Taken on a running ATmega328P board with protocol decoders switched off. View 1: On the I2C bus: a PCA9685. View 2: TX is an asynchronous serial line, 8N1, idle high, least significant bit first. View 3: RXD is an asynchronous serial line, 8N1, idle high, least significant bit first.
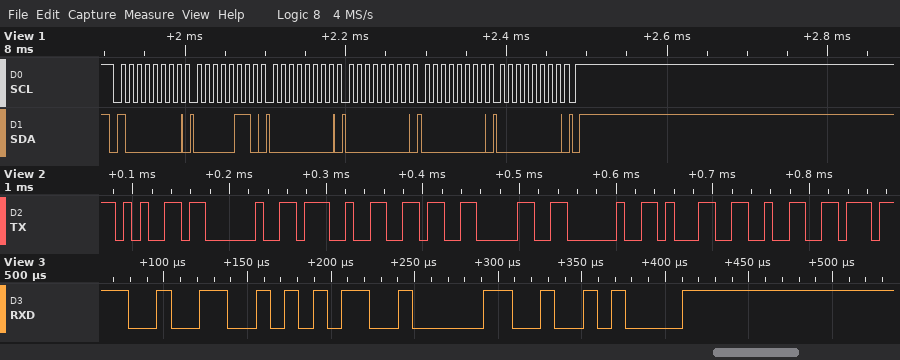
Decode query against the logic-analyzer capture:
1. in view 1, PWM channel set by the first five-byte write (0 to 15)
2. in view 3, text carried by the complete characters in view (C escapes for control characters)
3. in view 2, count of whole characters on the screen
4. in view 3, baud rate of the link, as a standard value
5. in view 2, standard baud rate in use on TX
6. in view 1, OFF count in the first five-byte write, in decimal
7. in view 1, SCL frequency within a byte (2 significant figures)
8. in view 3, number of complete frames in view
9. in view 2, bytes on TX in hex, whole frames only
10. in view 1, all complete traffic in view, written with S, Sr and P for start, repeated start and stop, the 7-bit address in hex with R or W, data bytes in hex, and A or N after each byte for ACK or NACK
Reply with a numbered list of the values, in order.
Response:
1. 0
2. "250\n"
3. 8
4. 115200 baud
5. 115200 baud
6. 0
7. 100 kHz
8. 4
9. 65 20 27 36 30 20 31 32
10. S 40W A 06 A 00 A 00 A 00 A 00 A P
